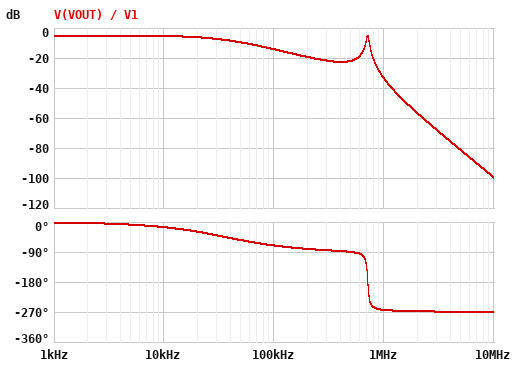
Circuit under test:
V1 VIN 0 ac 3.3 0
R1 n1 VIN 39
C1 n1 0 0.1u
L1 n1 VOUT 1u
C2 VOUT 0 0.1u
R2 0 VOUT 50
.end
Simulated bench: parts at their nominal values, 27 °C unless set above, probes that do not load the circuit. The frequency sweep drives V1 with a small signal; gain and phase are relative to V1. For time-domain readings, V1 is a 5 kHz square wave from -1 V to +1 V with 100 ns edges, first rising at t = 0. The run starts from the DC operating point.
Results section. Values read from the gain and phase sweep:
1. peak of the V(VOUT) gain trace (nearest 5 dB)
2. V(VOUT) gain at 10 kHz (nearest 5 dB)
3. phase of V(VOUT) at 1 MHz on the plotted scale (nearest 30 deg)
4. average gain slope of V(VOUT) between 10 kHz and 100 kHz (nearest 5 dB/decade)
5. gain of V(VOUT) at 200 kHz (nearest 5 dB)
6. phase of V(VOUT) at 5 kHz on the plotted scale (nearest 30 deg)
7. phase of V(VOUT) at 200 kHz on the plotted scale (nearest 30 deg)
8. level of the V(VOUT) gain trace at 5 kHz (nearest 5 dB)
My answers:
-5 dB
-5 dB
-270 deg
-10 dB/decade
-20 dB
0 deg
-90 deg
-5 dB
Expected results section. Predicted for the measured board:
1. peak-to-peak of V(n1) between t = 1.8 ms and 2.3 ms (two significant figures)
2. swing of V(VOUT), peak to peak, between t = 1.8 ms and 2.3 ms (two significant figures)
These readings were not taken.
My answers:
1.1 V
1.1 V
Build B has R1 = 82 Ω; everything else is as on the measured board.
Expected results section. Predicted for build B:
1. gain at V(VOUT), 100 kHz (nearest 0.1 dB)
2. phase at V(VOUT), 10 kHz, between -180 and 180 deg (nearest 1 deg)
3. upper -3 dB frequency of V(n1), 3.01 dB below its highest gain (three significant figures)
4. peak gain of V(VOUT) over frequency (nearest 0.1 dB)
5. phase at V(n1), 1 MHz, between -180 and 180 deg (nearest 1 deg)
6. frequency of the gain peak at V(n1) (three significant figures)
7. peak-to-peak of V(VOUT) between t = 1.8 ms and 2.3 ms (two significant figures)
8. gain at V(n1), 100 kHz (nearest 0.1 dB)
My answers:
-20.4 dB
-21 deg
726 kHz
-8.4 dB
-88 deg
712 kHz
760 mV
-20.7 dB
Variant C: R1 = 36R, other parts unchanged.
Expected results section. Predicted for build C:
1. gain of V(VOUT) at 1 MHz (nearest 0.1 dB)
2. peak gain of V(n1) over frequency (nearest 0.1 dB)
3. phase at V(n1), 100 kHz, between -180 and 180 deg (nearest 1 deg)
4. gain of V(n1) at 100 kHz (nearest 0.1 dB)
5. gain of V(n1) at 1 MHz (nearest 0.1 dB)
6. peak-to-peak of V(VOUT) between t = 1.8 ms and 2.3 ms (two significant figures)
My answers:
-32.9 dB
-4.7 dB
-69 deg
-13.9 dB
-23.5 dB
1.2 V
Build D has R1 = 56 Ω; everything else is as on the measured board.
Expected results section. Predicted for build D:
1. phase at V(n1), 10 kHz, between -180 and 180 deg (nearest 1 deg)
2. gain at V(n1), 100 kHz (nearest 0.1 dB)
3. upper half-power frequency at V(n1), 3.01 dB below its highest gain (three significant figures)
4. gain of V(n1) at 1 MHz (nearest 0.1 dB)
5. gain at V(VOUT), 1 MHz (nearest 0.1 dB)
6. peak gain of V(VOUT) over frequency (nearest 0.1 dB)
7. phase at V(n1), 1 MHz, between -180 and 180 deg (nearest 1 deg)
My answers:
-18 deg
-17.5 dB
728 kHz
-27.3 dB
-36.7 dB
-6.5 dB
-87 deg
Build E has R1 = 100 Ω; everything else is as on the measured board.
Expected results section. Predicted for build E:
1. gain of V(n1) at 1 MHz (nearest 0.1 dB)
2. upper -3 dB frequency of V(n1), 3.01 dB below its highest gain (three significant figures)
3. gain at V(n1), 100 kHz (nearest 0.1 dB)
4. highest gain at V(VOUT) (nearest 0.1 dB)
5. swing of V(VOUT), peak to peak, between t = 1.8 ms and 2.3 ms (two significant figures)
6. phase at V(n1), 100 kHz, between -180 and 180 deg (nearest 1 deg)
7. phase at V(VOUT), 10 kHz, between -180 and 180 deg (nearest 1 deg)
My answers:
-32.4 dB
725 kHz
-22.4 dB
-9.5 dB
670 mV
-76 deg
-23 deg
